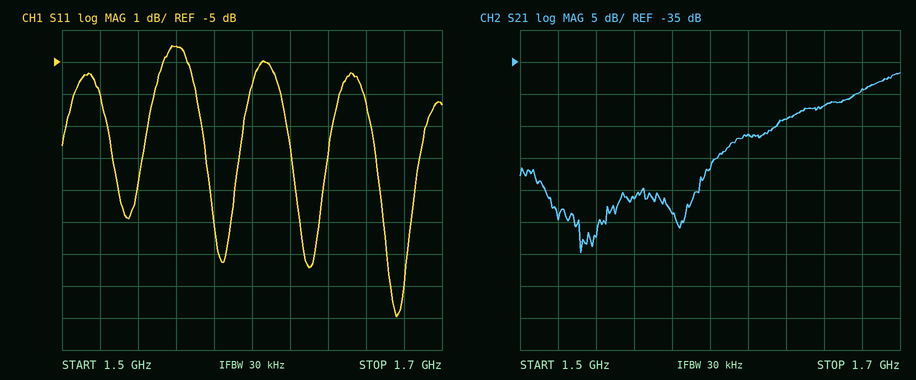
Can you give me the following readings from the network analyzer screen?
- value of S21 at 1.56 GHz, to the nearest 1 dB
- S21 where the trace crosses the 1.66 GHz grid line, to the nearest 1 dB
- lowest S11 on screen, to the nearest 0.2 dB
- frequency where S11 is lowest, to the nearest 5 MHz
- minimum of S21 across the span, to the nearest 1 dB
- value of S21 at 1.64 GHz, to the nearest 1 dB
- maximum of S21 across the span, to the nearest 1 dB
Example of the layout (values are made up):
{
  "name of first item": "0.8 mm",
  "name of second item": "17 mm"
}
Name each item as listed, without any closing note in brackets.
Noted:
{
  "value of S21 at 1.56 GHz, to the nearest 1 dB": "-56 dB",
  "S21 where the trace crosses the 1.66 GHz grid line, to the nearest 1 dB": "-42 dB",
  "lowest S11 on screen, to the nearest 0.2 dB": "-13.0 dB",
  "frequency where S11 is lowest, to the nearest 5 MHz": "1.675 GHz",
  "minimum of S21 across the span, to the nearest 1 dB": "-65 dB",
  "value of S21 at 1.64 GHz, to the nearest 1 dB": "-44 dB",
  "maximum of S21 across the span, to the nearest 1 dB": "-37 dB"
}
